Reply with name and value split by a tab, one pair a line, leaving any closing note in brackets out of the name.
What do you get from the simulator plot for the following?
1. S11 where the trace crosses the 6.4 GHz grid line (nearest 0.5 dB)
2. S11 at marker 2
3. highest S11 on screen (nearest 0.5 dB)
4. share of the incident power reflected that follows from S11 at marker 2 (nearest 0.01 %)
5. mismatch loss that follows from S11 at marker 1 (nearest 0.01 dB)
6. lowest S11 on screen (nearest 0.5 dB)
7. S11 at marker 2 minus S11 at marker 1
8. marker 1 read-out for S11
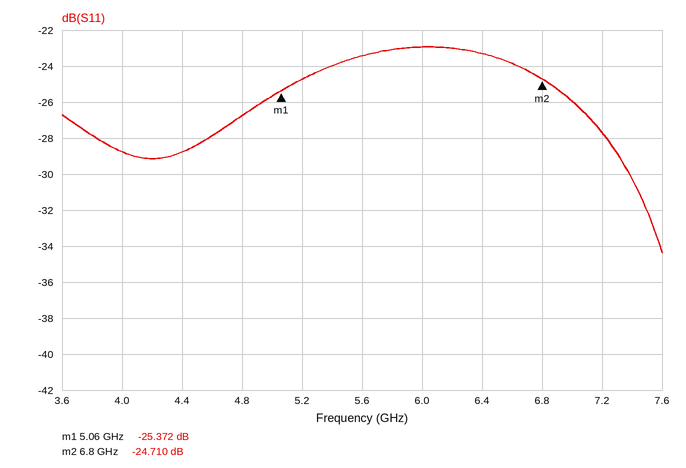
S11 where the trace crosses the 6.4 GHz grid line	-23.5 dB
S11 at marker 2	-24.710 dB
highest S11 on screen	-23.0 dB
share of the incident power reflected that follows from S11 at marker 2	0.34 %
mismatch loss that follows from S11 at marker 1	0.01 dB
lowest S11 on screen	-34.5 dB
S11 at marker 2 minus S11 at marker 1	0.662 dB
marker 1 read-out for S11	-25.372 dB
